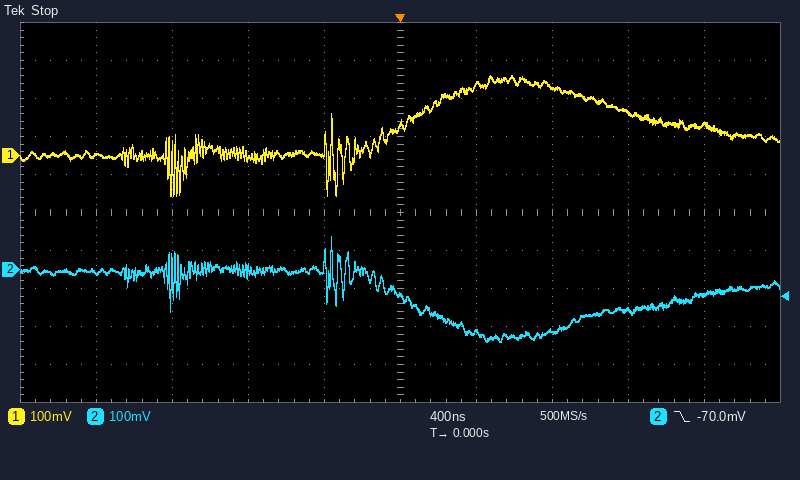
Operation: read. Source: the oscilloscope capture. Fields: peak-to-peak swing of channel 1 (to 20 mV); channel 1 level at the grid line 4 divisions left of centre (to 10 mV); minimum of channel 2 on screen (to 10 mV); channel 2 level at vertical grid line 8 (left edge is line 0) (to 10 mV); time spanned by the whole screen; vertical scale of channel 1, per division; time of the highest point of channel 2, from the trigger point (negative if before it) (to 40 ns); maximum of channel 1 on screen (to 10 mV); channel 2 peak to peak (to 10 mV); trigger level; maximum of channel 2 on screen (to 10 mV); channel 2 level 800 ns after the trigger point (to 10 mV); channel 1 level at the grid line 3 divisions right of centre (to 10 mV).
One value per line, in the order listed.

320 mV
0 mV
-190 mV
-110 mV
4 µs
100 mV
-360 ns
210 mV
280 mV
-70.0 mV
90 mV
-160 mV
110 mV
